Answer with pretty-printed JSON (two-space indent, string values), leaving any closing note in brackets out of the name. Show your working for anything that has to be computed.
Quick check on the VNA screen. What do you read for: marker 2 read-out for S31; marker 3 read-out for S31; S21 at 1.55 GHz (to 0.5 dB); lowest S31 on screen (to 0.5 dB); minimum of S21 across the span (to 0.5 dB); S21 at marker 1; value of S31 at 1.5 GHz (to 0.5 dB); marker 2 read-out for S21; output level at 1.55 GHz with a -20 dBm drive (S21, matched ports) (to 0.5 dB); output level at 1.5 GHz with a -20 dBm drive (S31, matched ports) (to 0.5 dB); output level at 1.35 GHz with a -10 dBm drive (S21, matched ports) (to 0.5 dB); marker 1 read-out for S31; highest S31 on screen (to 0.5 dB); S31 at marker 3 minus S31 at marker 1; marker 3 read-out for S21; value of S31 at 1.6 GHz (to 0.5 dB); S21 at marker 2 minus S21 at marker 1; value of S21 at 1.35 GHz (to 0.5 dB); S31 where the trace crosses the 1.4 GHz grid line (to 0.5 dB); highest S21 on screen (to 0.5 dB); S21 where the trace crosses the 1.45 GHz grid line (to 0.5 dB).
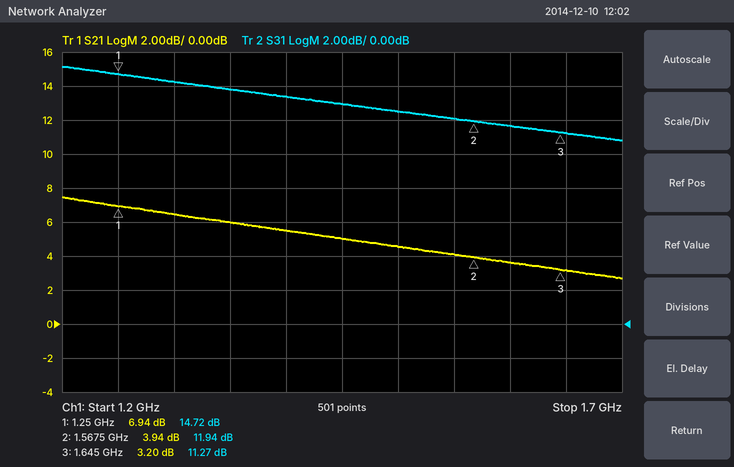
{
  "marker 2 read-out for S31": "11.94 dB",
  "marker 3 read-out for S31": "11.27 dB",
  "S21 at 1.55 GHz": "4.0 dB",
  "lowest S31 on screen": "11.0 dB",
  "minimum of S21 across the span": "2.5 dB",
  "S21 at marker 1": "6.94 dB",
  "value of S31 at 1.5 GHz": "12.5 dB",
  "marker 2 read-out for S21": "3.94 dB",
  "output level at 1.55 GHz with a -20 dBm drive (S21, matched ports)": "-20 dBm + (4.0 dB) = -16.0 dBm",
  "output level at 1.5 GHz with a -20 dBm drive (S31, matched ports)": "-20 dBm + (12.5 dB) = -7.5 dBm",
  "output level at 1.35 GHz with a -10 dBm drive (S21, matched ports)": "-10 dBm + (6.0 dB) = -4.0 dBm",
  "marker 1 read-out for S31": "14.72 dB",
  "highest S31 on screen": "15.0 dB",
  "S31 at marker 3 minus S31 at marker 1": "11.27 − (14.72) = -3.45 dB",
  "marker 3 read-out for S21": "3.20 dB",
  "value of S31 at 1.6 GHz": "11.5 dB",
  "S21 at marker 2 minus S21 at marker 1": "3.94 − (6.94) = -3.00 dB",
  "value of S21 at 1.35 GHz": "6.0 dB",
  "S31 where the trace crosses the 1.4 GHz grid line": "13.5 dB",
  "highest S21 on screen": "7.5 dB",
  "S21 where the trace crosses the 1.45 GHz grid line": "5.0 dB"
}
